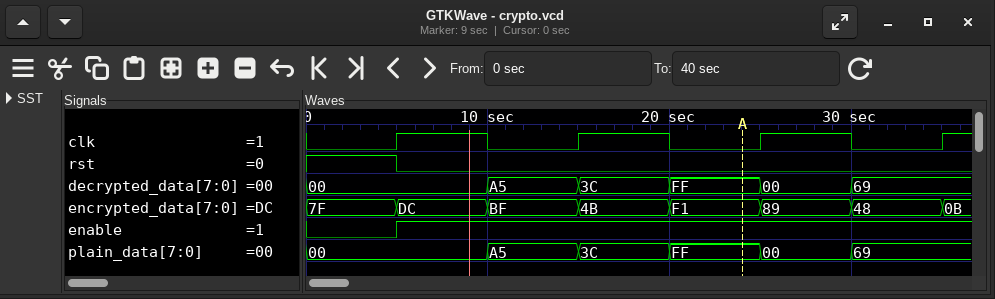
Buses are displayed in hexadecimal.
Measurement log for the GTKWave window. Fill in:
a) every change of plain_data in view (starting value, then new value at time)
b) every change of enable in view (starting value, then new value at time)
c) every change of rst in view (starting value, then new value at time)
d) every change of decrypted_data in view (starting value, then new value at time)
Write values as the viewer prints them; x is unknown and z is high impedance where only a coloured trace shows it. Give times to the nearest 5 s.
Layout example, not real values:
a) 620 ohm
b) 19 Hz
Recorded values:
a) 00, A5 at 10 s, 3C at 15 s, FF at 20 s, 00 at 25 s, 69 at 30 s
b) 0, 1 at 5 s
c) 1, 0 at 5 s
d) 00, A5 at 10 s, 3C at 15 s, FF at 20 s, 00 at 25 s, 69 at 30 s
